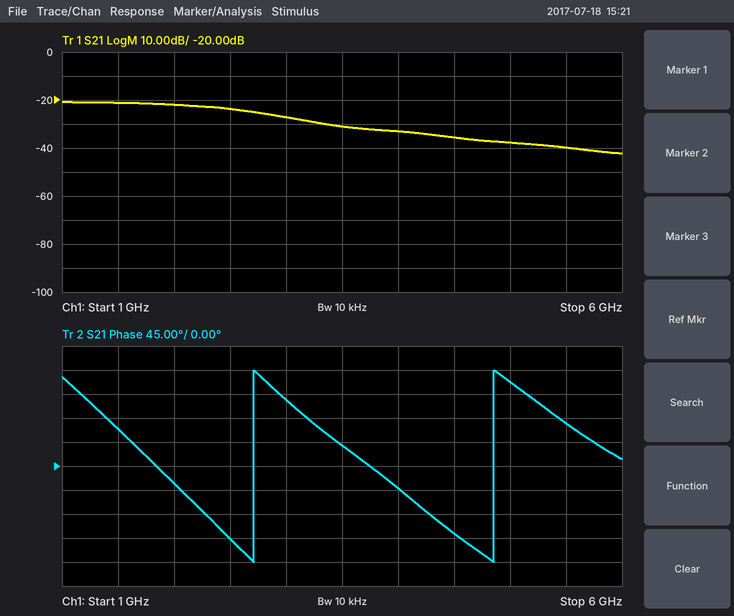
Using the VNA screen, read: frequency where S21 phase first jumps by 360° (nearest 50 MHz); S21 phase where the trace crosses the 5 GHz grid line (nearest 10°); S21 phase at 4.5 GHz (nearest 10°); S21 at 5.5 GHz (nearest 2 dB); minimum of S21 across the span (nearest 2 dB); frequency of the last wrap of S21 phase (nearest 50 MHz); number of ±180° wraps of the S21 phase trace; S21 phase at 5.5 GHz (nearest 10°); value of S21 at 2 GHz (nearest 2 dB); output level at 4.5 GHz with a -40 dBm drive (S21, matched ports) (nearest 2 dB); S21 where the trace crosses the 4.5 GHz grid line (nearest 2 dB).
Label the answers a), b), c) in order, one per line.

a) 2.70 GHz
b) 160°
c) -130°
d) -40 dB
e) -42 dB
f) 4.85 GHz
g) 2
h) 80°
i) -22 dB
j) -76 dBm
k) -36 dB
